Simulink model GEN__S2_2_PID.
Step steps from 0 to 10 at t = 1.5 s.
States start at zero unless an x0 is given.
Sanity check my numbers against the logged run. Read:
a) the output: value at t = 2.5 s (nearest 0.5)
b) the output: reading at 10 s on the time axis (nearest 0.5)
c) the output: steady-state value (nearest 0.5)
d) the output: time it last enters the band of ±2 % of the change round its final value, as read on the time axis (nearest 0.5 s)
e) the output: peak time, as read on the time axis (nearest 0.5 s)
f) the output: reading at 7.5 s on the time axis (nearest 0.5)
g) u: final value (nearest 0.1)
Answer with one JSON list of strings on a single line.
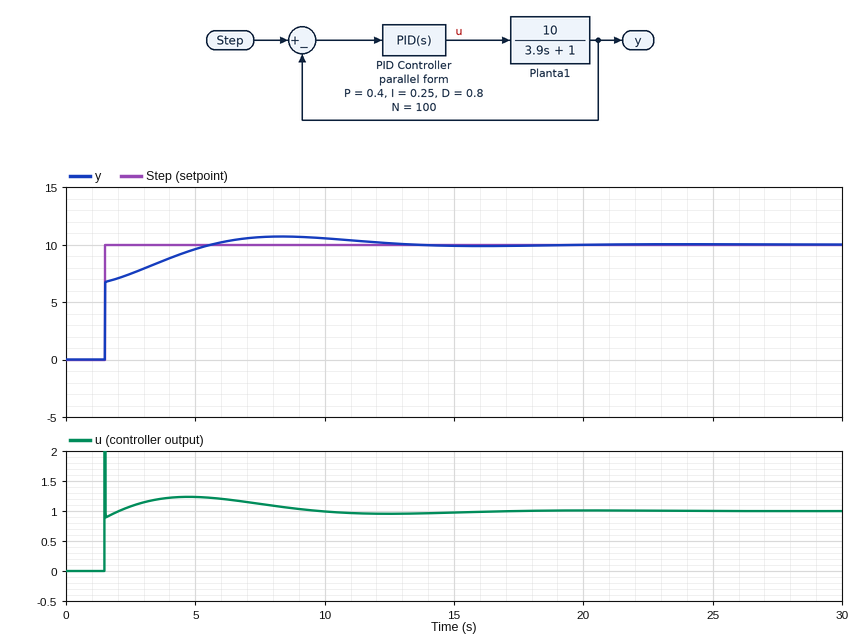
["7.5", "10.5", "10.0", "12.0 s", "8.5 s", "10.5", "1.0"]
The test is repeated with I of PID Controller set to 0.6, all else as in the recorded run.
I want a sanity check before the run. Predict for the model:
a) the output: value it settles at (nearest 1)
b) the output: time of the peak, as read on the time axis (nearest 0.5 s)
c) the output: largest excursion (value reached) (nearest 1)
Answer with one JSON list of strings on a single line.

["10", "6.0 s", "11"]
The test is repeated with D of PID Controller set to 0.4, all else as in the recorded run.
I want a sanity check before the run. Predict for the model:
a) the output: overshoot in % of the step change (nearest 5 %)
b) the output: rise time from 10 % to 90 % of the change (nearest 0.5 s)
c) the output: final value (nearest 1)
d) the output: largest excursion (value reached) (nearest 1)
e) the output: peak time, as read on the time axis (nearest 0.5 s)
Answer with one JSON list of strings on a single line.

["10 %", "2.0 s", "10", "11", "6.5 s"]
